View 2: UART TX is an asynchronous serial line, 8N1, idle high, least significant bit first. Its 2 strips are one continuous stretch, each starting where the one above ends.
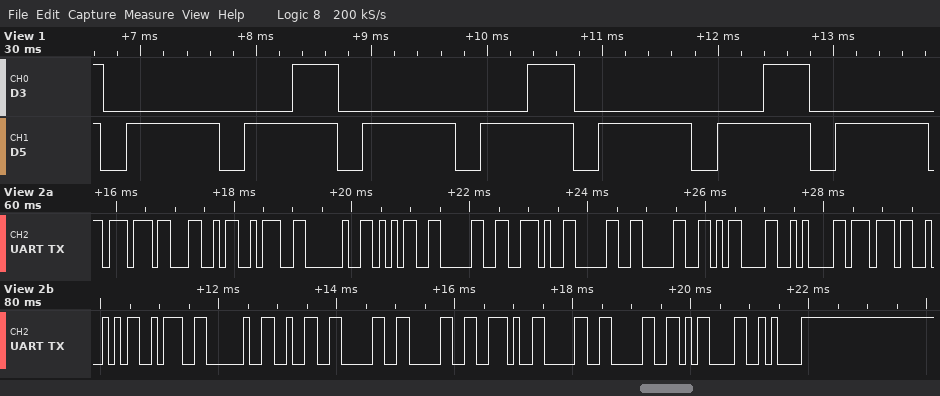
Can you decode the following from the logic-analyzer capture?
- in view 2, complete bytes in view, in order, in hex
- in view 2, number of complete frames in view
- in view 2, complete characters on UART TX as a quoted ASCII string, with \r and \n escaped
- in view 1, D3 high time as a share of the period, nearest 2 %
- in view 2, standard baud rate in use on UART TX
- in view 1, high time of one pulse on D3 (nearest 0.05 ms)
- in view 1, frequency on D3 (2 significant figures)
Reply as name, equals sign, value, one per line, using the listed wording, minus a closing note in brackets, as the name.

in view 2, complete bytes in view, in order, in hex = 77 4C 3A 20 35 30 2E 30 30 0D 0A 77 52 3A 20 32 30 30 2E 30 30 0D 0A
in view 2, number of complete frames in view = 23
in view 2, complete characters on UART TX as a quoted ASCII string, with \r and \n escaped = "wL: 50.00\r\nwR: 200.00\r\n"
in view 1, D3 high time as a share of the period, nearest 2 % = 20 %
in view 2, standard baud rate in use on UART TX = 9600 baud
in view 1, high time of one pulse on D3 = 0.40 ms
in view 1, frequency on D3 = 490 Hz
